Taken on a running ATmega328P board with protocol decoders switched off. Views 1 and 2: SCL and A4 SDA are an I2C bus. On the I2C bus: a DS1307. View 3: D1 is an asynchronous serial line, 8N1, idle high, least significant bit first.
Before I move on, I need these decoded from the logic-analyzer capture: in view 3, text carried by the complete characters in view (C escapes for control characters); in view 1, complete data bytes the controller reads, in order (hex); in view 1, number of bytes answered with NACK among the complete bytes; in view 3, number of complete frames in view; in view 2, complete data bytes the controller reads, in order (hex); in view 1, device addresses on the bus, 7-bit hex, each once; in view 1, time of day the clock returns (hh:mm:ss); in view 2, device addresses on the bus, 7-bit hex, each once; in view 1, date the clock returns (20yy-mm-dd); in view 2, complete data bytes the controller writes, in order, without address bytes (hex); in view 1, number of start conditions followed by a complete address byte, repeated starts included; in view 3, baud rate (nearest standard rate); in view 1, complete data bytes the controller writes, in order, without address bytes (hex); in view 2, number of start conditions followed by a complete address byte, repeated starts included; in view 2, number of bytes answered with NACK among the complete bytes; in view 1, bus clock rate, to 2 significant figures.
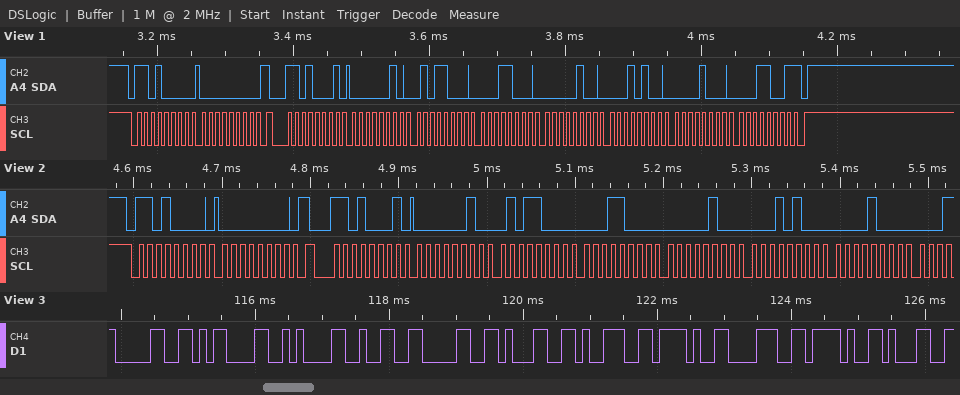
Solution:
"0\r\n2019/8/1"
02 58 18 04 14 08 19
1
11
02 58 18 04 14 08
0x68
18:58:02
0x68
2019-08-14
00
2
9600 baud
00
2
0
100 kHz
